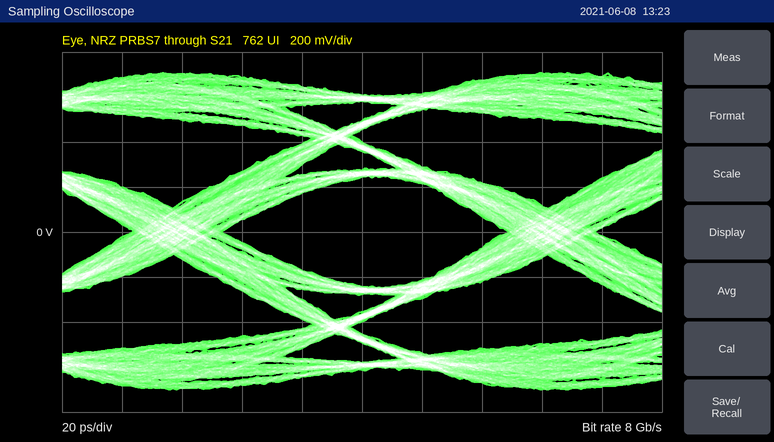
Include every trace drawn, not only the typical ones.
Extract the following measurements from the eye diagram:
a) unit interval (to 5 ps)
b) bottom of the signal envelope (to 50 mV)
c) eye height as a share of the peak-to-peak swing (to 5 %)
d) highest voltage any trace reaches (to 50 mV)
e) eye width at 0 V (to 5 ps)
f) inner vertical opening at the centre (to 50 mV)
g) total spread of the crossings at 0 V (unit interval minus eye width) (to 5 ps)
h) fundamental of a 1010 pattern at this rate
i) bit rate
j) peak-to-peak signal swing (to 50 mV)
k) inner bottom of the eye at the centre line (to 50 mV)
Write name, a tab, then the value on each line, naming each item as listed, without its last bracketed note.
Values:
unit interval	125 ps
bottom of the signal envelope	-700 mV
eye height as a share of the peak-to-peak swing	35 %
highest voltage any trace reaches	700 mV
eye width at 0 V	95 ps
inner vertical opening at the centre	500 mV
total spread of the crossings at 0 V (unit interval minus eye width)	30 ps
fundamental of a 1010 pattern at this rate	4 GHz
bit rate	8 Gb/s
peak-to-peak signal swing	1.40 V
inner bottom of the eye at the centre line	-250 mV
